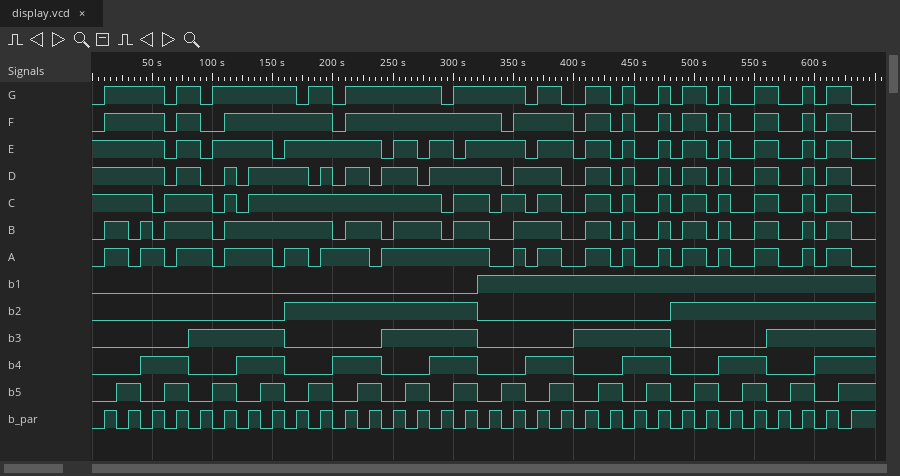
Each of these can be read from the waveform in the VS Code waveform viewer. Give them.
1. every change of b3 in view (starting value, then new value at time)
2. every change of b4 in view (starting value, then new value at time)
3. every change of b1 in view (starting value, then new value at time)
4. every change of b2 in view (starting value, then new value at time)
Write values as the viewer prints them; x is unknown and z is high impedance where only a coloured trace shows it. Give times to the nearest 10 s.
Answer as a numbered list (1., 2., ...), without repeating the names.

1. 0, 1 at 80 s, 0 at 160 s, 1 at 240 s, 0 at 320 s, 1 at 400 s, 0 at 480 s, 1 at 560 s
2. 0, 1 at 40 s, 0 at 80 s, 1 at 120 s, 0 at 160 s, 1 at 200 s, 0 at 240 s, 1 at 280 s, 0 at 320 s, 1 at 360 s, 0 at 400 s, 1 at 440 s, 0 at 480 s, 1 at 520 s, 0 at 560 s, 1 at 600 s
3. 0, 1 at 320 s
4. 0, 1 at 160 s, 0 at 320 s, 1 at 480 s
